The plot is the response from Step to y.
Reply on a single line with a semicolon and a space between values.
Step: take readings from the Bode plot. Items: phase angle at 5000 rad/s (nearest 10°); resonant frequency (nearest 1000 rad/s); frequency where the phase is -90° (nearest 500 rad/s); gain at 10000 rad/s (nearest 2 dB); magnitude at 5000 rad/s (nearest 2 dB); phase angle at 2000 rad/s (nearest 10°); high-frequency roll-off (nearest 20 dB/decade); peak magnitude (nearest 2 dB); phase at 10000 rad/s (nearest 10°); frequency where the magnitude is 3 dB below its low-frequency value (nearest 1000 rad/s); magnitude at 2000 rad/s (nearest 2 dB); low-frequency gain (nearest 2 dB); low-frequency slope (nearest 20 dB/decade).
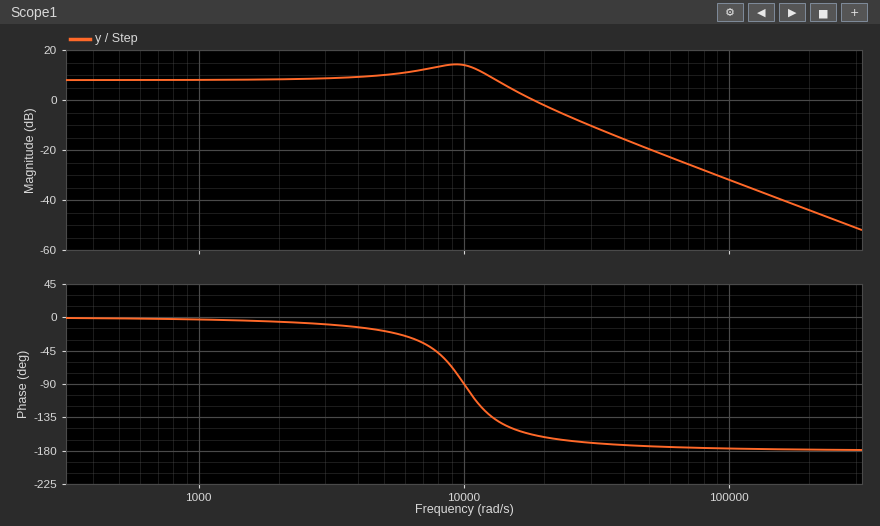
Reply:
-20°; 9000 rad/s; 10000 rad/s; 14 dB; 10 dB; -10°; -40 dB/decade; 14 dB; -90°; 15000 rad/s; 8 dB; 8 dB; 0 dB/decade
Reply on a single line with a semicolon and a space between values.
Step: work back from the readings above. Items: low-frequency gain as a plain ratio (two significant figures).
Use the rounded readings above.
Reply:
2.5
